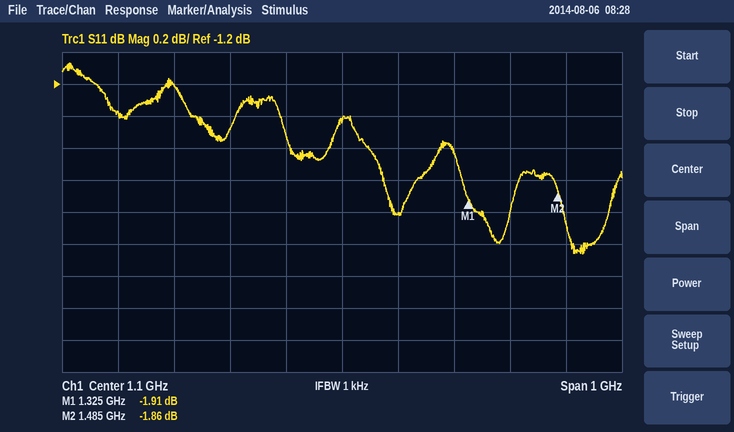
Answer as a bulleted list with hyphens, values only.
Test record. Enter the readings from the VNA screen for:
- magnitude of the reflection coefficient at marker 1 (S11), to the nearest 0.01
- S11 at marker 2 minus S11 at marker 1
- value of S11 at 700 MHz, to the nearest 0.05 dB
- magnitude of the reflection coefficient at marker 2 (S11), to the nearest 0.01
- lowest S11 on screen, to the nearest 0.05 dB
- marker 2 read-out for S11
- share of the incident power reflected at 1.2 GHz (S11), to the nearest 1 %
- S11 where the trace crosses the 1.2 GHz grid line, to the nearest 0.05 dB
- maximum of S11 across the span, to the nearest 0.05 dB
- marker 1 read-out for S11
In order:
- 0.80
- 0.05 dB
- -1.40 dB
- 0.81
- -2.25 dB
- -1.86 dB
- 63 %
- -2.00 dB
- -1.05 dB
- -1.91 dB
